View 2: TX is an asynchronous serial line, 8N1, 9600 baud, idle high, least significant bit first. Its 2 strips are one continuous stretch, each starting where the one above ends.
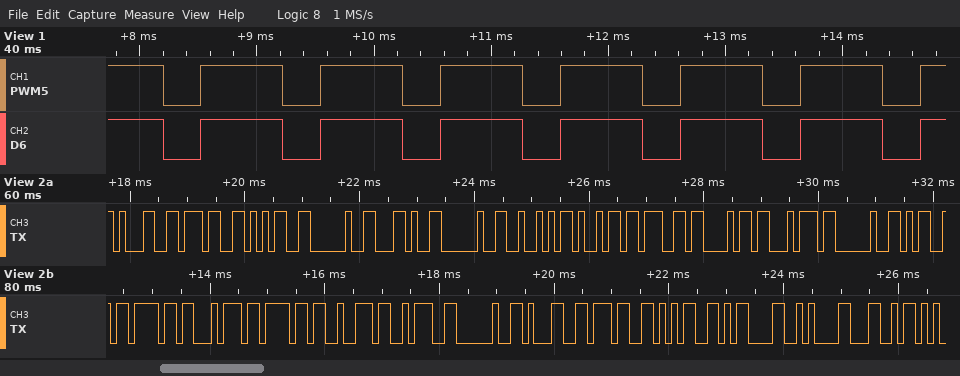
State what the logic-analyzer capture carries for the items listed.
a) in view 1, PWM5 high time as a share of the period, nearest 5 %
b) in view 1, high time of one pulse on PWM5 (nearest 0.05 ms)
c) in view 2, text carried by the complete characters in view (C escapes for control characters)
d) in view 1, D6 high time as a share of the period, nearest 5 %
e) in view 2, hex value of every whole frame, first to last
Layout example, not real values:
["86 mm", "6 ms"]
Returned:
["70 %", "0.70 ms", "\"175 , Right Motor: 175\\r\\nL\"", "70 %", "31 37 35 20 2C 20 52 69 67 68 74 20 4D 6F 74 6F 72 3A 20 31 37 35 0D 0A 4C"]
